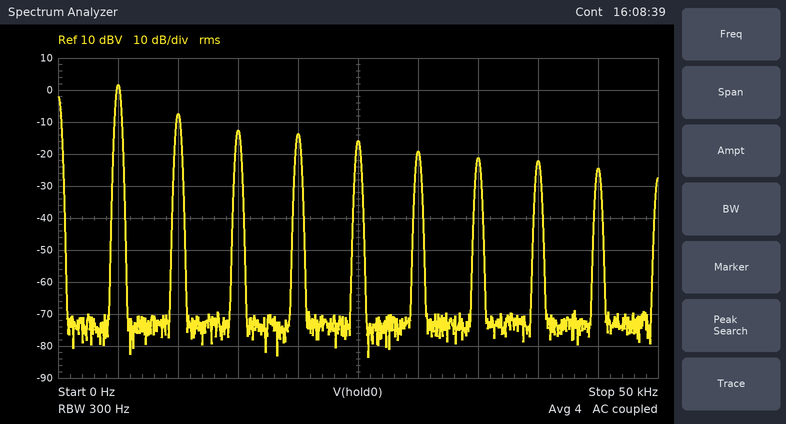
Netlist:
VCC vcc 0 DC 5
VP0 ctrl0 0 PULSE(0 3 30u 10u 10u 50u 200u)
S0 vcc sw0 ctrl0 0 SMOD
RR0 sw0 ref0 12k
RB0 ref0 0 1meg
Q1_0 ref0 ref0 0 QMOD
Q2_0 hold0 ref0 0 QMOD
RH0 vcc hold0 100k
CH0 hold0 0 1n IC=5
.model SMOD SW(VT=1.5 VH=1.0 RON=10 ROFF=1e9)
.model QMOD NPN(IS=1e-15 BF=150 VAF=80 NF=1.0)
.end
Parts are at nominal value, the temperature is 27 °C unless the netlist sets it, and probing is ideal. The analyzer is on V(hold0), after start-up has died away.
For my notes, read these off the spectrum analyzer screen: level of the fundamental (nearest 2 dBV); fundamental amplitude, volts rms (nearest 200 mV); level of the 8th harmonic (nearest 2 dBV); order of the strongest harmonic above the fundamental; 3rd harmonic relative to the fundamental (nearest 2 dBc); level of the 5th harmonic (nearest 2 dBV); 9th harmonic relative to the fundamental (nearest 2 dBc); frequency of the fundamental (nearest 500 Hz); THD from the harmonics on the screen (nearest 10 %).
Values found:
2 dBV
1.2 V
-22 dBV
2
-14 dBc
-16 dBV
-26 dBc
5.0 kHz
50 %
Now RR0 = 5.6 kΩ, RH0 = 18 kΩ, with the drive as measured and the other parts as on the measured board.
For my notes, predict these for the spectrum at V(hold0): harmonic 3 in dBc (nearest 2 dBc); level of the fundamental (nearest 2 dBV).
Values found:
-20 dBc
6 dBV
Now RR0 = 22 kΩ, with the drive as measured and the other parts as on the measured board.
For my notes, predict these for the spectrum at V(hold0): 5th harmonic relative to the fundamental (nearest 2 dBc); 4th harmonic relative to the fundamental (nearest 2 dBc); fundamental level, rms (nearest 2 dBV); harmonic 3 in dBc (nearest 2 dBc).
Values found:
-20 dBc
-18 dBc
2 dBV
-16 dBc
